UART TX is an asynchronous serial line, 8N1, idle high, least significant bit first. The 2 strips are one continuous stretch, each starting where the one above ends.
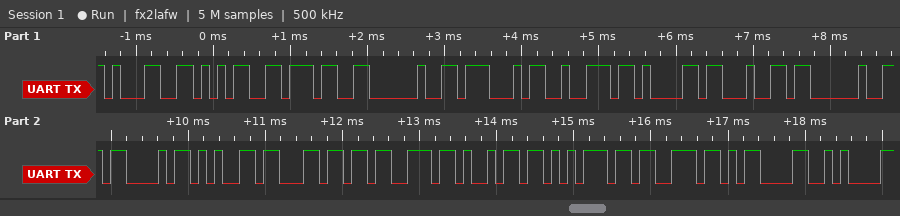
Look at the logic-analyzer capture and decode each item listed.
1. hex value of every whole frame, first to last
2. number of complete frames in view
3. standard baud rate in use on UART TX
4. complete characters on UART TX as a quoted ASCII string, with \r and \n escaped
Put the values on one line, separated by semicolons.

31 35 37 20 47 72 61 64 20 43 65 6C 73 69 75 73 0D 0A; 18; 9600 baud; "157 Grad Celsius\r\n"
